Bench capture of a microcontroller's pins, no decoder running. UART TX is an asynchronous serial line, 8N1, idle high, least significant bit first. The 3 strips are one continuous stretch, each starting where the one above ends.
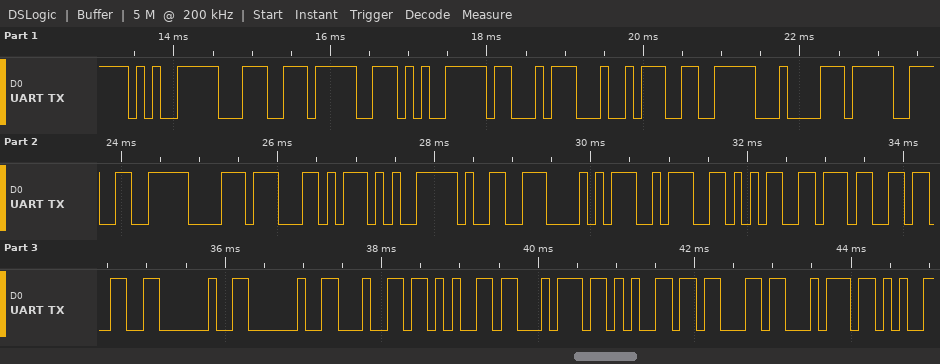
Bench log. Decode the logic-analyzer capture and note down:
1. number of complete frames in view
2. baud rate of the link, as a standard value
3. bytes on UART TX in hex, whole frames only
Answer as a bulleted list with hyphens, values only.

- 27
- 9600 baud
- E5 9C 9F E5 A3 A4 E6 84 9F E6 B8 AC E5 99 A8 3A 35 37 33 20 20 64 65 74 65 63 74
